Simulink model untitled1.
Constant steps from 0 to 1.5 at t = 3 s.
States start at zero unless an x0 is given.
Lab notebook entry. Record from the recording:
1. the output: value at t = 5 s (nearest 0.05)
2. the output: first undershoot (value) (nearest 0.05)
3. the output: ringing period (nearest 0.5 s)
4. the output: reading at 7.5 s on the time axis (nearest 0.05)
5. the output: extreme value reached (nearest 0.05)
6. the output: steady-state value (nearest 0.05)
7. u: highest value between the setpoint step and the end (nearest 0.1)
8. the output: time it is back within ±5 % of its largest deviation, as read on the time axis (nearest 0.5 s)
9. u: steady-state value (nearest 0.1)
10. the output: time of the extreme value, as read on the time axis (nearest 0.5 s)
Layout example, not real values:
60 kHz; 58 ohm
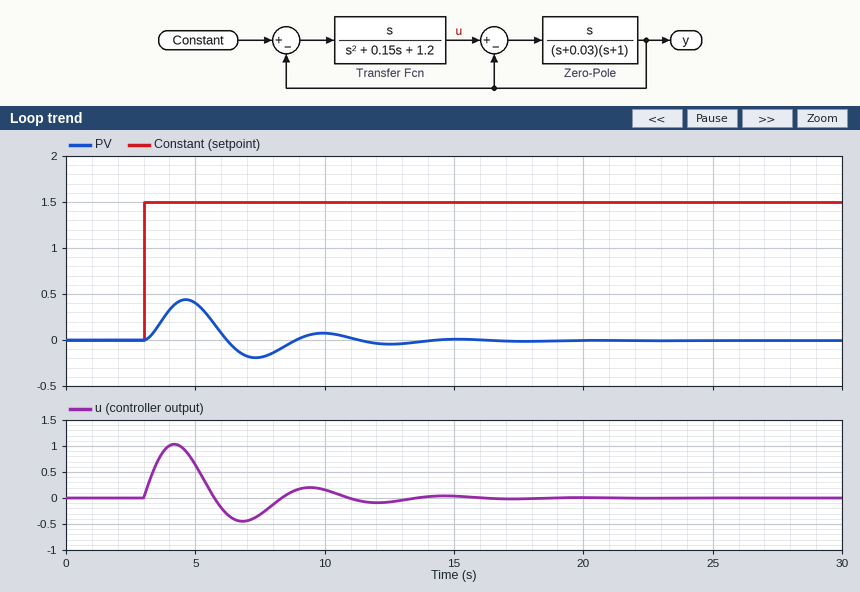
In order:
0.40; -0.20; 5.5 s; -0.20; 0.45; 0.00; 1.0; 13.5 s; 0.0; 4.5 s
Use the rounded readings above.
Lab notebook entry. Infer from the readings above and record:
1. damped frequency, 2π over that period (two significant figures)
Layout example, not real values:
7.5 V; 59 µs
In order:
1.1 rad/s
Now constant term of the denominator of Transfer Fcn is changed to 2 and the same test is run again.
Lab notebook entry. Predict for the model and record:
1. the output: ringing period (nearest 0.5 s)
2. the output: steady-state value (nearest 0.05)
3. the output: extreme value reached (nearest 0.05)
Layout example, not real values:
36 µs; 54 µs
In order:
4.0 s; 0.00; 0.35
